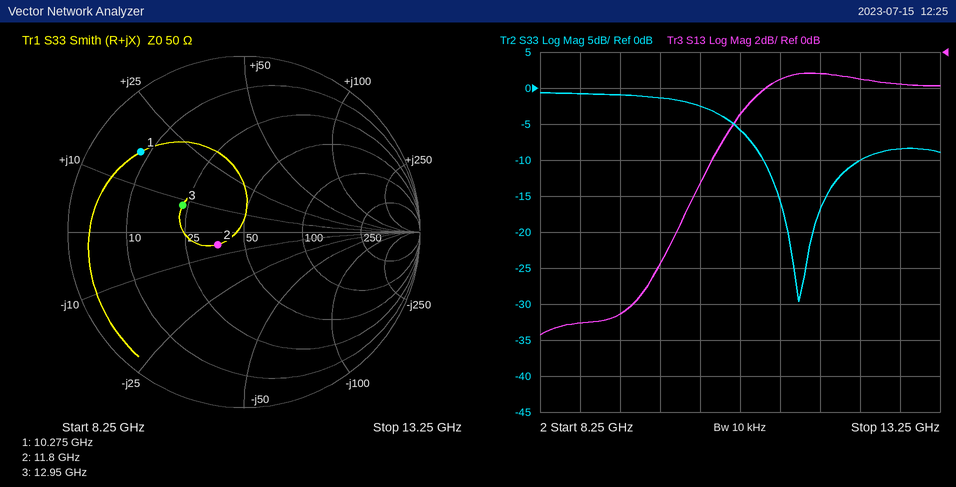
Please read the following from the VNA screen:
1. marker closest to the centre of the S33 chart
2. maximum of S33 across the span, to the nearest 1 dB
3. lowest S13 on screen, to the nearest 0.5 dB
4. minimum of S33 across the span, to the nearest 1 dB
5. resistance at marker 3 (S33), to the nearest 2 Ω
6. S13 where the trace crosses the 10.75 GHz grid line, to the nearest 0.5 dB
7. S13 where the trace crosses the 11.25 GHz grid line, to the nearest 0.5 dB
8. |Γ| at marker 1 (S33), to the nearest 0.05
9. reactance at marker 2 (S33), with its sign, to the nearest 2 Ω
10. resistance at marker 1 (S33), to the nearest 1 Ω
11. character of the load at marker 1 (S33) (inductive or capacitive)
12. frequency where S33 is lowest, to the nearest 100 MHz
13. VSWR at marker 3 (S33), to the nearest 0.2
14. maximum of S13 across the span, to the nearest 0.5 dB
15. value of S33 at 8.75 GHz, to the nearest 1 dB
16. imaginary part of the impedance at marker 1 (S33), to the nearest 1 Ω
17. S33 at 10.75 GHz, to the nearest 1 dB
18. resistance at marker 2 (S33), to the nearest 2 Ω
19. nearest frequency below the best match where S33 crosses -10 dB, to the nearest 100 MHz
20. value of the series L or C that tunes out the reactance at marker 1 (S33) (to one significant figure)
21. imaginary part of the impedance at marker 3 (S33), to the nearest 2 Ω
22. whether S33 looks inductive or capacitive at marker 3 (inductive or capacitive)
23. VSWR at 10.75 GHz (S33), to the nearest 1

marker 2
-1 dB
-15.5 dB
-30 dB
24 Ω
-3.5 dB
-1.5 dB
0.75
-6 Ω
8 Ω
inductive
11.5 GHz
2.2
-1.0 dB
-1 dB
+17 Ω
-6 dB
36 Ω
11.0 GHz
900 fF
+8 Ω
inductive
3
